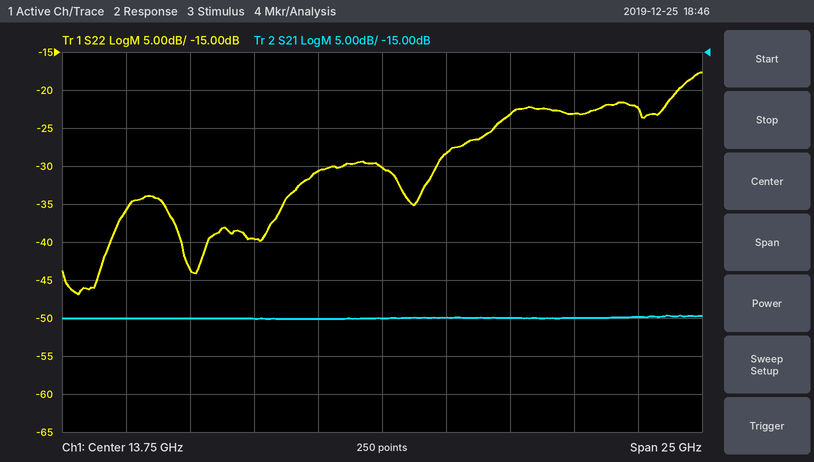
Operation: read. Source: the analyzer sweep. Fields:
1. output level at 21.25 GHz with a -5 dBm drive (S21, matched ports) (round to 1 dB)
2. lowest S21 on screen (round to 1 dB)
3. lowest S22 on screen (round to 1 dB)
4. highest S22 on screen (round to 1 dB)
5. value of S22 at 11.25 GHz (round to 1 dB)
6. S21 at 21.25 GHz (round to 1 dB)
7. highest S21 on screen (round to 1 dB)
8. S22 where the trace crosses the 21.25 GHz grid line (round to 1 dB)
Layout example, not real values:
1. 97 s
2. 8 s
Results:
1. -55 dBm
2. -50 dB
3. -47 dB
4. -18 dB
5. -31 dB
6. -50 dB
7. -50 dB
8. -23 dB
